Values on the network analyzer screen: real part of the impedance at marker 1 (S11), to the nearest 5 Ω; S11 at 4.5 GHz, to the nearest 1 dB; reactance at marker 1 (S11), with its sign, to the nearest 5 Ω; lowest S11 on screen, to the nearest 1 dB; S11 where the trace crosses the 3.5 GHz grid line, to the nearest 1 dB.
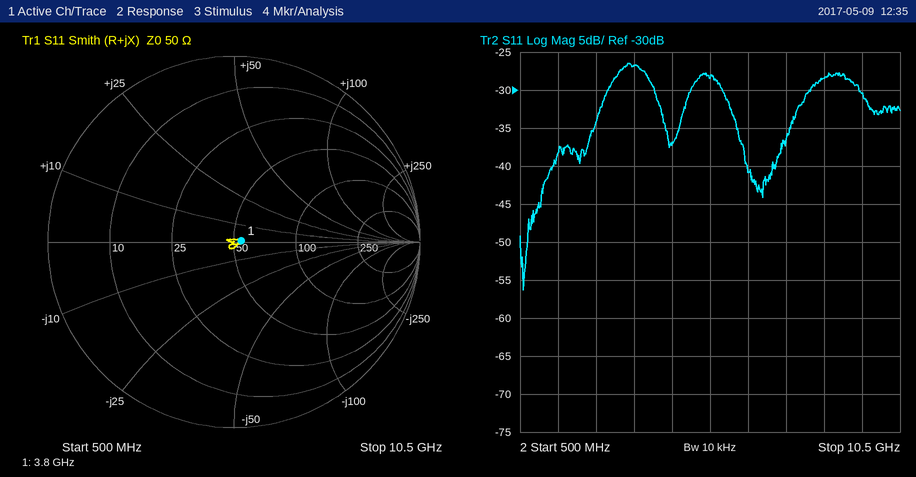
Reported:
55 Ω
-37 dB
0 Ω
-56 dB
-27 dB
